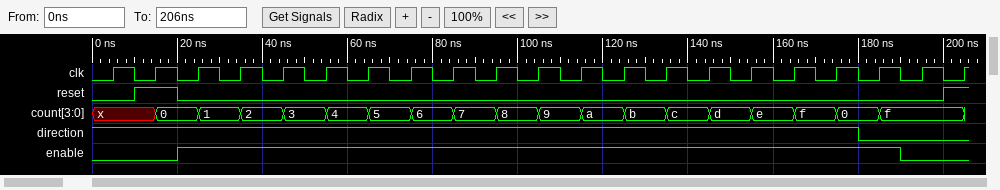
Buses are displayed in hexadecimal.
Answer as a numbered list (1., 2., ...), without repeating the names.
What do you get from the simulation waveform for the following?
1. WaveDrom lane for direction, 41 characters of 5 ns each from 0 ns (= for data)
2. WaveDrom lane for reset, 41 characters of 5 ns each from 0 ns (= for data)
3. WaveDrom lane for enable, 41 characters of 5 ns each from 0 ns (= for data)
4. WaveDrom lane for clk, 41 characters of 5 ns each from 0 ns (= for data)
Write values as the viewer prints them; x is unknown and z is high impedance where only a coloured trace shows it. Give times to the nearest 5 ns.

1. {name: 'direction', wave: '1...................................0....'}
2. {name: 'reset', wave: '0.1.0...................................1'}
3. {name: 'enable', wave: '0...1.................................0..'}
4. {name: 'clk', wave: '01010101010101010101010101010101010101010'}
